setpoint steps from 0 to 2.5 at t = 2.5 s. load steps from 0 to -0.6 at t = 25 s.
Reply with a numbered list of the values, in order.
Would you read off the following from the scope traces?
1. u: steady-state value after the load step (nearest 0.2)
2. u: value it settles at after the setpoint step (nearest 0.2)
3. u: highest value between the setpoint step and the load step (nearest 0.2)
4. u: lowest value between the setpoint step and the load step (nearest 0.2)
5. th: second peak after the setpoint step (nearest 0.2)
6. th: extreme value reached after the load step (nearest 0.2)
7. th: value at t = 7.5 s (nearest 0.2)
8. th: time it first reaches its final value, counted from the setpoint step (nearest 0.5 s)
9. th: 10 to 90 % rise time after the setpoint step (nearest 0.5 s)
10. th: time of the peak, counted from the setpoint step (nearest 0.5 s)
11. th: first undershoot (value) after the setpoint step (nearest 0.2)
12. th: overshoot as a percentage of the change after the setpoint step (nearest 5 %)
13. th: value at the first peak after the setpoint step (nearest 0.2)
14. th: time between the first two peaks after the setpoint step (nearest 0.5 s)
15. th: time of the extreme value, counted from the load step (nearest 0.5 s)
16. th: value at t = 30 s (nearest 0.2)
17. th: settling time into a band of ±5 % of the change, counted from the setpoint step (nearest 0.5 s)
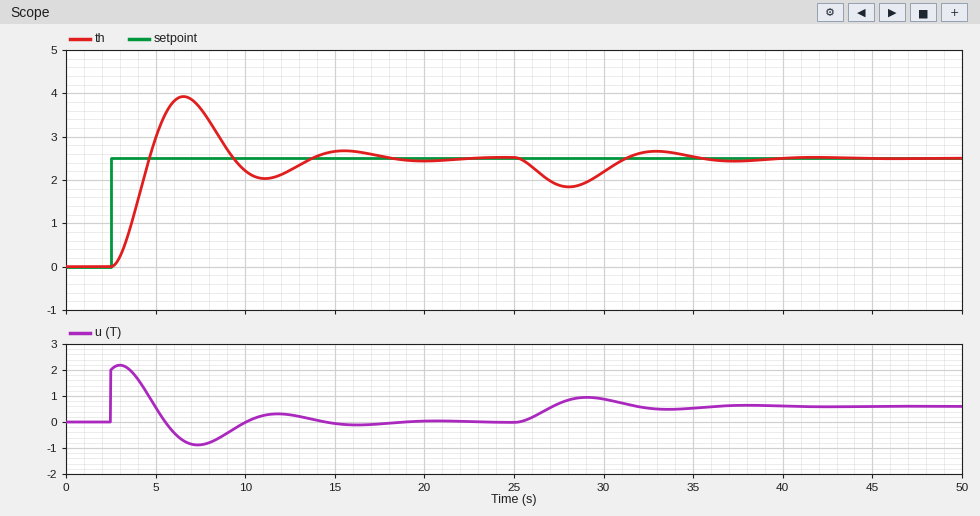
1. 0.6
2. 0.0
3. 2.2
4. -0.8
5. 2.6
6. 1.8
7. 3.6
8. 2.0 s
9. 1.5 s
10. 4.0 s
11. 2.0
12. 55 %
13. 4.0
14. 9.0 s
15. 3.0 s
16. 2.2
17. 14.0 s
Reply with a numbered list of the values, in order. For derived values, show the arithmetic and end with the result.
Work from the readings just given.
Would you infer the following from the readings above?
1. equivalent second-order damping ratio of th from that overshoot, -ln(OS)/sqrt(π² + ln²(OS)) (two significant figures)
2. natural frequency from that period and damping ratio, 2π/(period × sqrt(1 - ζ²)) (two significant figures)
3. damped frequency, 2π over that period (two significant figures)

1. ln(0.55) = -0.598; 0.598 / sqrt(9.870 + 0.357) = 0.19
2. 2π / (9 × sqrt(1 - 0.19²)) = 0.71 rad/s
3. 2π / 9 = 0.70 rad/s
